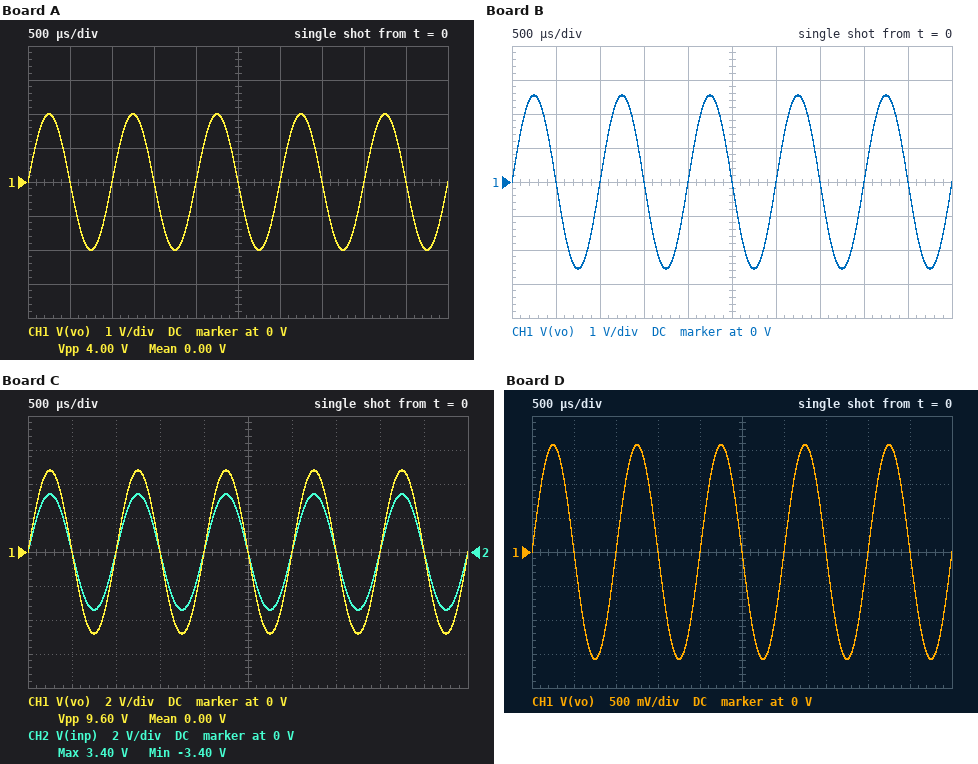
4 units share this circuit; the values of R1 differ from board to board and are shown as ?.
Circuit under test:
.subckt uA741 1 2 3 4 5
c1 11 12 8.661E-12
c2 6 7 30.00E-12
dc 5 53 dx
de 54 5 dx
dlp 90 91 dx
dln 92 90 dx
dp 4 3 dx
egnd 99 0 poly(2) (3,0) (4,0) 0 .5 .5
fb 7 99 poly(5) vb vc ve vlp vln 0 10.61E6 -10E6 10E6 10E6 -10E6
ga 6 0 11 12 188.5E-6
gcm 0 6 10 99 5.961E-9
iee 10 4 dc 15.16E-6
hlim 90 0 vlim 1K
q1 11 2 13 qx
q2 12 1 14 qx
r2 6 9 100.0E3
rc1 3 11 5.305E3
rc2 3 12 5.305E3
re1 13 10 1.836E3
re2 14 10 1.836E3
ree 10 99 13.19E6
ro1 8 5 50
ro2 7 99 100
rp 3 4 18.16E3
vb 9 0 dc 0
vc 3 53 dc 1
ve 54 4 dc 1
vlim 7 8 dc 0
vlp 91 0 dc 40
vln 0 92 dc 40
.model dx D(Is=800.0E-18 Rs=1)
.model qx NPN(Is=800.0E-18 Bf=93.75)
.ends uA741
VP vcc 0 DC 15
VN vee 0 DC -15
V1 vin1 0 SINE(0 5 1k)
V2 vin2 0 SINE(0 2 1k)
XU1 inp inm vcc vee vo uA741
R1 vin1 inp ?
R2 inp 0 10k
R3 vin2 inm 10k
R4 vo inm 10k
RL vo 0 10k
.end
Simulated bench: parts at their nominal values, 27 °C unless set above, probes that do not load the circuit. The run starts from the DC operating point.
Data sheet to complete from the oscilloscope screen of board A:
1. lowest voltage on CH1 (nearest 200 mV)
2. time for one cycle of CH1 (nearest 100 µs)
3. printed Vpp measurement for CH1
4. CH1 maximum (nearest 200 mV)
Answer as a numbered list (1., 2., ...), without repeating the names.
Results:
1. -2.0 V
2. 1.0 ms
3. 4.00 V
4. 2.0 V
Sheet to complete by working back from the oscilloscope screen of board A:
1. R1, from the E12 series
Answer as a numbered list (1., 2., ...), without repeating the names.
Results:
1. 15 kΩ
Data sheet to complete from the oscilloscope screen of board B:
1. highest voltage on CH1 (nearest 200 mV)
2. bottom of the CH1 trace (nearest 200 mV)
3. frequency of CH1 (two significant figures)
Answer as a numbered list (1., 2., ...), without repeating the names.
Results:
1. 2.6 V
2. -2.6 V
3. 1.0 kHz
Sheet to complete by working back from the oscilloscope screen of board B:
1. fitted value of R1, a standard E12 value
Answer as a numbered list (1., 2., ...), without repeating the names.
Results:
1. 12 kΩ
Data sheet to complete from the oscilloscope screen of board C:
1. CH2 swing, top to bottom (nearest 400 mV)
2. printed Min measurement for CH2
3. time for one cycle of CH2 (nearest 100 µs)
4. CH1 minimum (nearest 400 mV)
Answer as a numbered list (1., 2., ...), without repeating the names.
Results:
1. 6.8 V
2. -3.40 V
3. 1.0 ms
4. -4.8 V
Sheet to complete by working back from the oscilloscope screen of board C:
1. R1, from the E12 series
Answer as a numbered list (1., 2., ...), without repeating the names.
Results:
1. 4.7 kΩ
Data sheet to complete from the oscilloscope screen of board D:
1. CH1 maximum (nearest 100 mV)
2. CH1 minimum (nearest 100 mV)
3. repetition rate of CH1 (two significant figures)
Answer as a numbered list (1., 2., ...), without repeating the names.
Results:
1. 1.6 V
2. -1.6 V
3. 1.0 kHz
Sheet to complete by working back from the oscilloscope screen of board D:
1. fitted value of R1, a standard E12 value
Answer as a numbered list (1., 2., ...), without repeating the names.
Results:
1. 18 kΩ
